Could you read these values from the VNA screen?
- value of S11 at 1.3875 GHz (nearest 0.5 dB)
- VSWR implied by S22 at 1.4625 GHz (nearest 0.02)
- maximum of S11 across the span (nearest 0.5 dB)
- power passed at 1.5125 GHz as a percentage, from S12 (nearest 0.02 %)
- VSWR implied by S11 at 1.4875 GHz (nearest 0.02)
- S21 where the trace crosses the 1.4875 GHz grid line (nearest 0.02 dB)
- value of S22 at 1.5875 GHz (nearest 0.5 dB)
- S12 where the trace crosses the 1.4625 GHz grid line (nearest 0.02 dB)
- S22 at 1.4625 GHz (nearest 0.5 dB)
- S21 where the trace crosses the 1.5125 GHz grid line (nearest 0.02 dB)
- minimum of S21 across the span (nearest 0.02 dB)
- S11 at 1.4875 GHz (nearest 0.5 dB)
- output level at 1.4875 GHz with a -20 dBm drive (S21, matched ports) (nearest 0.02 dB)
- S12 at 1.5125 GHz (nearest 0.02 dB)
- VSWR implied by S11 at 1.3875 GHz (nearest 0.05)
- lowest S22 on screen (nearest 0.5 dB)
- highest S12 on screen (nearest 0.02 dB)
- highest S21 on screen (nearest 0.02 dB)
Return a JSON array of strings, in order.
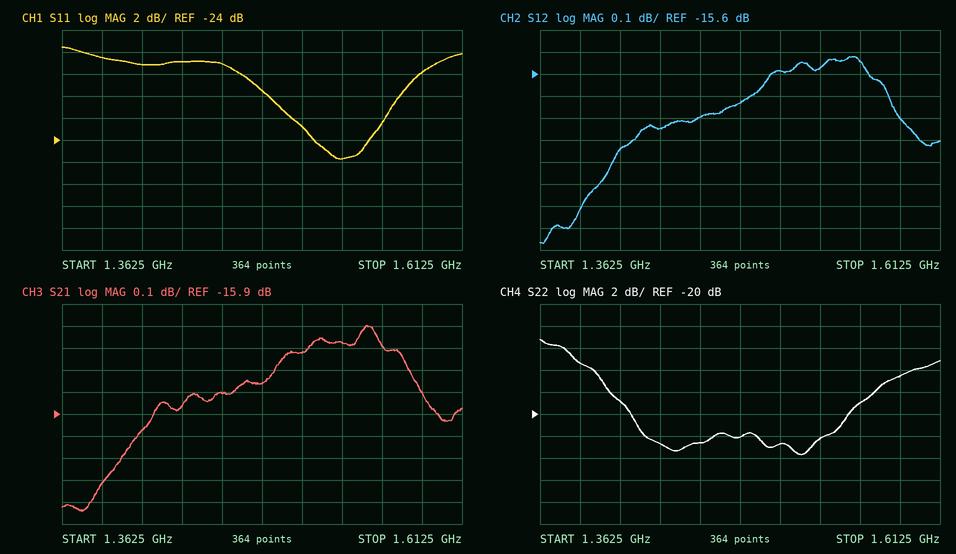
["-16.5 dB", "1.16", "-15.5 dB", "2.76 %", "1.24", "-15.76 dB", "-16.5 dB", "-15.80 dB", "-22.5 dB", "-15.62 dB", "-16.34 dB", "-19.5 dB", "-35.76 dBm", "-15.58 dB", "1.35", "-23.5 dB", "-15.52 dB", "-15.50 dB"]
